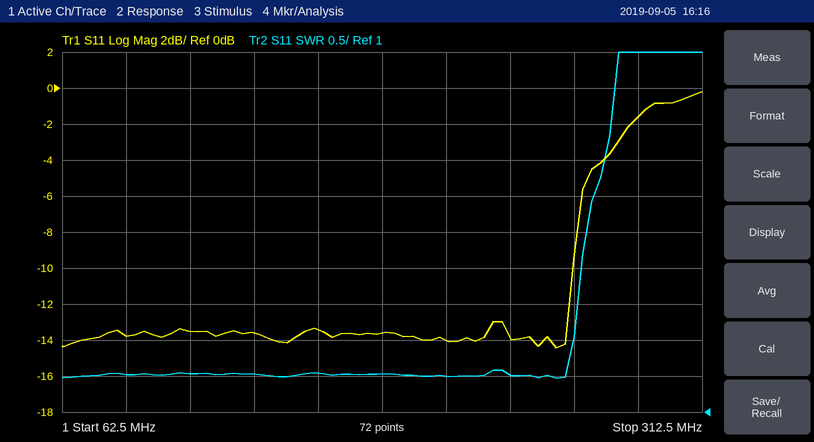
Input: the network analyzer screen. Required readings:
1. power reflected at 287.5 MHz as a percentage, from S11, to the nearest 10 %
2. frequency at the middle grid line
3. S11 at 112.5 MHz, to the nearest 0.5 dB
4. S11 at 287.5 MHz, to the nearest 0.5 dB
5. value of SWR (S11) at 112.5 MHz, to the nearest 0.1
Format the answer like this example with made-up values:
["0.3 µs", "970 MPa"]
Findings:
["70 %", "187.5 MHz", "-13.5 dB", "-1.5 dB", "1.5"]
